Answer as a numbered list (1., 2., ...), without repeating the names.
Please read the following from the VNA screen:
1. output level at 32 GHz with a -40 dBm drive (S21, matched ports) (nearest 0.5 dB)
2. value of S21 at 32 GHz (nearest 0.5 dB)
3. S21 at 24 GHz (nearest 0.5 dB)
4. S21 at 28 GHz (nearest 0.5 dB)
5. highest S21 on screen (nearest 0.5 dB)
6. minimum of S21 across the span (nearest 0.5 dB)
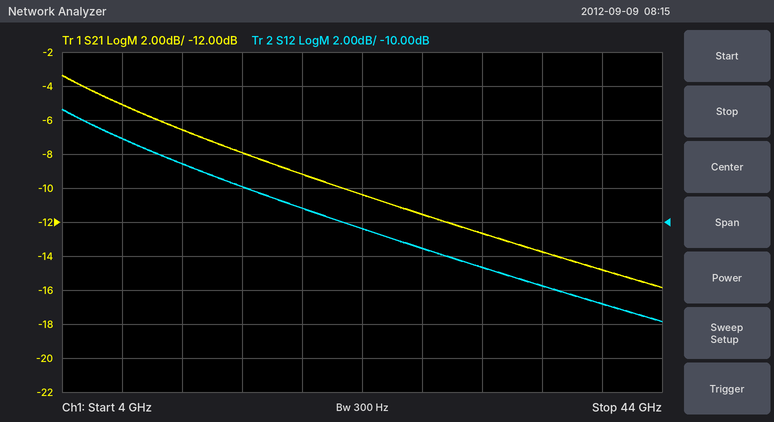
1. -52.5 dBm
2. -12.5 dB
3. -10.5 dB
4. -11.5 dB
5. -3.5 dB
6. -16.0 dB
